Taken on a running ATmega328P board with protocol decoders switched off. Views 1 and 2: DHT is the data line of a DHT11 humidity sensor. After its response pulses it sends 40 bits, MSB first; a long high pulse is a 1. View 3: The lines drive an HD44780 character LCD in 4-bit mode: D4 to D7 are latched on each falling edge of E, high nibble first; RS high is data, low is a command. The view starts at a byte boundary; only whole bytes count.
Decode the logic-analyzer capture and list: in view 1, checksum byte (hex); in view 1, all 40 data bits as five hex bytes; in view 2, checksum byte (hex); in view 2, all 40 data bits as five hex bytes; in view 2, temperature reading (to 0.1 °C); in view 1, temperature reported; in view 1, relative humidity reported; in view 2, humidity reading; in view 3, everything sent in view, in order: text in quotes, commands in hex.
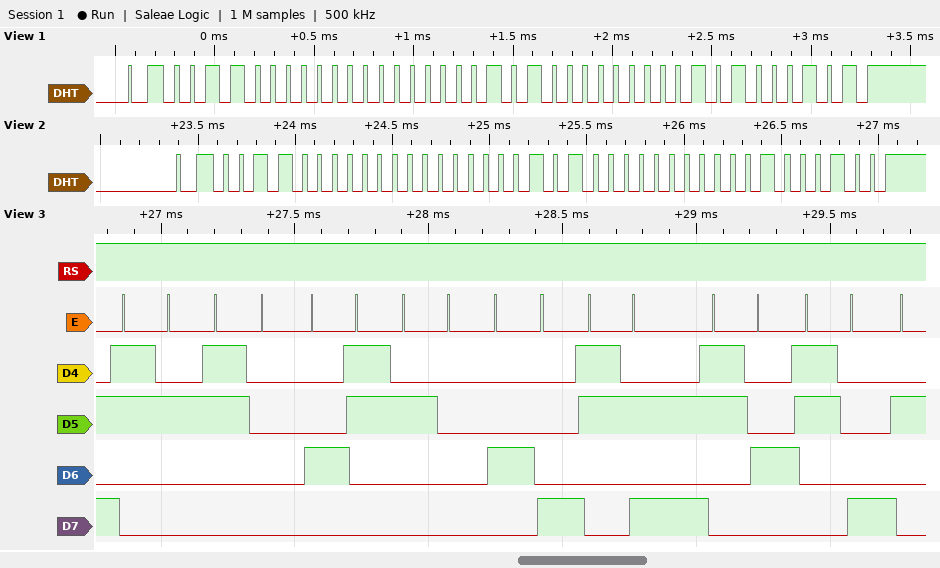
0x45
30 00 14 01 45
0x44
30 00 14 00 44
20.0 °C
20.1 °C
48 %
48 %
"20C H:48"
